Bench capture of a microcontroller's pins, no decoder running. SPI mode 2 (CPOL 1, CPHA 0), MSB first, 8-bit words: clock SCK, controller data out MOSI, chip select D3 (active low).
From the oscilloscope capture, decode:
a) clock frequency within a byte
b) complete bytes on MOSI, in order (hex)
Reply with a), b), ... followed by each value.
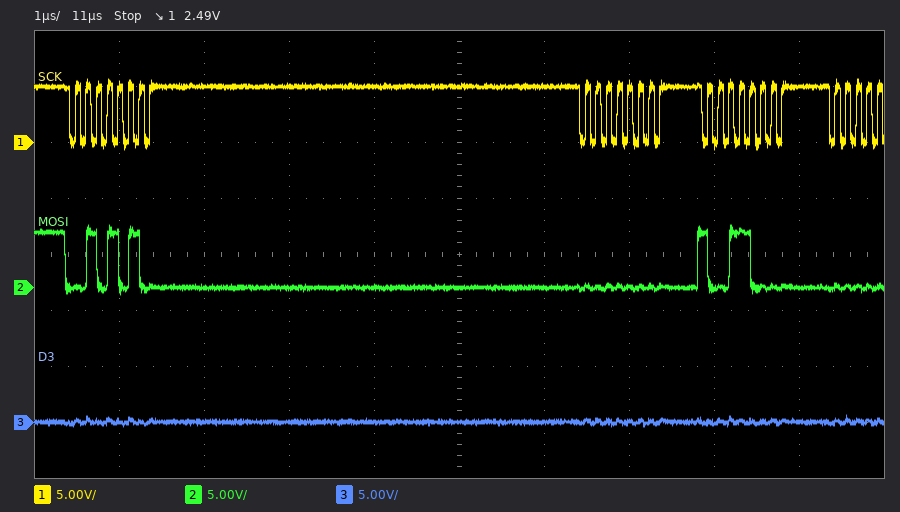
a) 8 MHz
b) 2A 00 98
